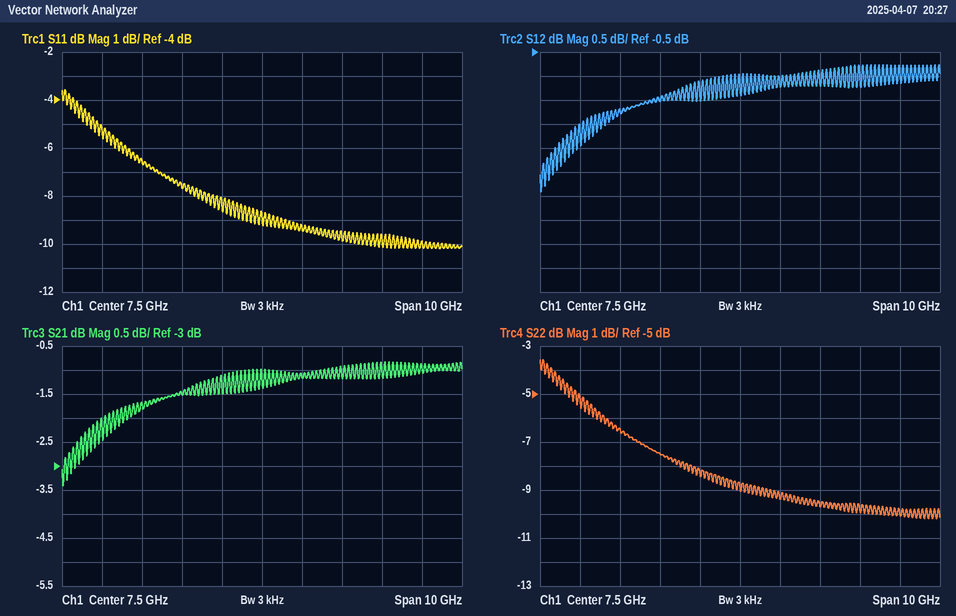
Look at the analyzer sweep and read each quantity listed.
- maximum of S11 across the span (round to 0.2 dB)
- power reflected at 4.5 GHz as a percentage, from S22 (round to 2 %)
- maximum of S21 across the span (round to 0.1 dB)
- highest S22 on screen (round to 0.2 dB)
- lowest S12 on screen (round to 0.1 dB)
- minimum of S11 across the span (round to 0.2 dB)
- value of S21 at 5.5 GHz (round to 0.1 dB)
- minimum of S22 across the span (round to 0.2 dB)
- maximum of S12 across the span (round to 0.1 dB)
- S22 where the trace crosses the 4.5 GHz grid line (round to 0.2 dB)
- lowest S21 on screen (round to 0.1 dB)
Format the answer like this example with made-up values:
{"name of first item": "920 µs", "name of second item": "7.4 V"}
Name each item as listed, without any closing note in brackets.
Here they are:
{"maximum of S11 across the span": "-3.6 dB", "power reflected at 4.5 GHz as a percentage, from S22": "22 %", "maximum of S21 across the span": "-0.8 dB", "highest S22 on screen": "-3.6 dB", "lowest S12 on screen": "-3.4 dB", "minimum of S11 across the span": "-10.2 dB", "value of S21 at 5.5 GHz": "-1.5 dB", "minimum of S22 across the span": "-10.2 dB", "maximum of S12 across the span": "-0.8 dB", "S22 where the trace crosses the 4.5 GHz grid line": "-6.4 dB", "lowest S21 on screen": "-3.4 dB"}
